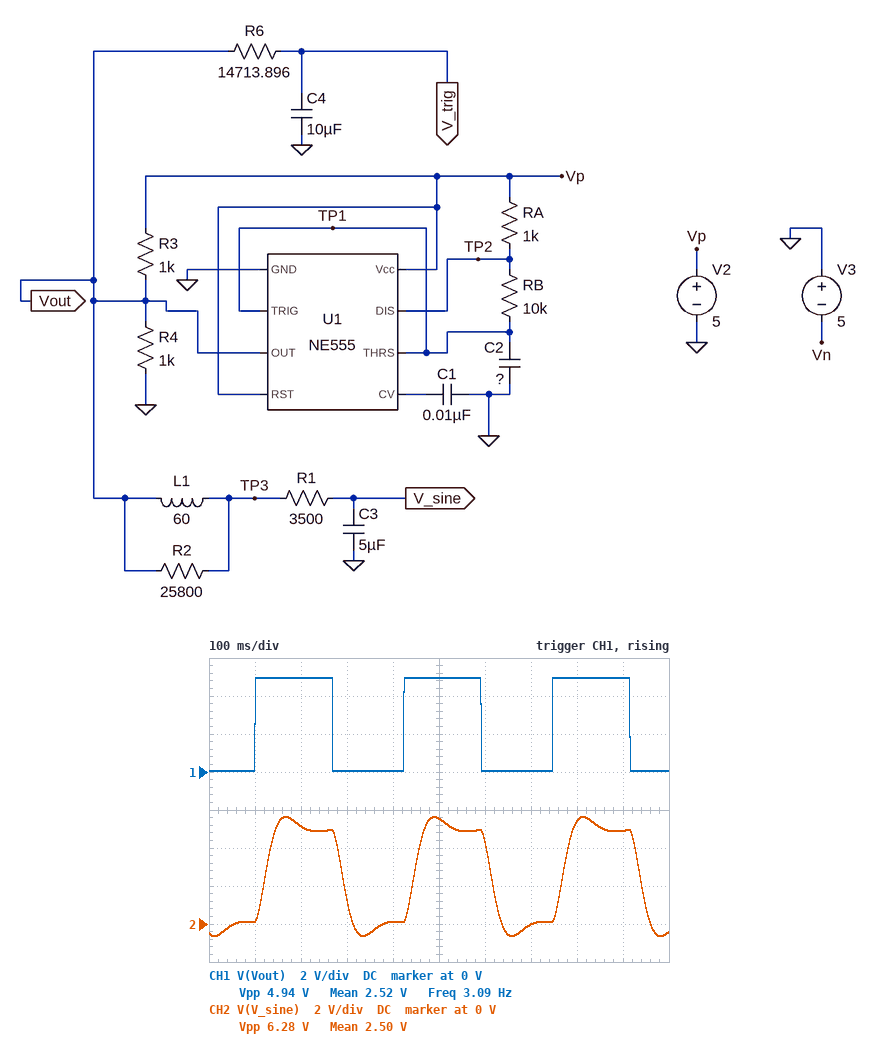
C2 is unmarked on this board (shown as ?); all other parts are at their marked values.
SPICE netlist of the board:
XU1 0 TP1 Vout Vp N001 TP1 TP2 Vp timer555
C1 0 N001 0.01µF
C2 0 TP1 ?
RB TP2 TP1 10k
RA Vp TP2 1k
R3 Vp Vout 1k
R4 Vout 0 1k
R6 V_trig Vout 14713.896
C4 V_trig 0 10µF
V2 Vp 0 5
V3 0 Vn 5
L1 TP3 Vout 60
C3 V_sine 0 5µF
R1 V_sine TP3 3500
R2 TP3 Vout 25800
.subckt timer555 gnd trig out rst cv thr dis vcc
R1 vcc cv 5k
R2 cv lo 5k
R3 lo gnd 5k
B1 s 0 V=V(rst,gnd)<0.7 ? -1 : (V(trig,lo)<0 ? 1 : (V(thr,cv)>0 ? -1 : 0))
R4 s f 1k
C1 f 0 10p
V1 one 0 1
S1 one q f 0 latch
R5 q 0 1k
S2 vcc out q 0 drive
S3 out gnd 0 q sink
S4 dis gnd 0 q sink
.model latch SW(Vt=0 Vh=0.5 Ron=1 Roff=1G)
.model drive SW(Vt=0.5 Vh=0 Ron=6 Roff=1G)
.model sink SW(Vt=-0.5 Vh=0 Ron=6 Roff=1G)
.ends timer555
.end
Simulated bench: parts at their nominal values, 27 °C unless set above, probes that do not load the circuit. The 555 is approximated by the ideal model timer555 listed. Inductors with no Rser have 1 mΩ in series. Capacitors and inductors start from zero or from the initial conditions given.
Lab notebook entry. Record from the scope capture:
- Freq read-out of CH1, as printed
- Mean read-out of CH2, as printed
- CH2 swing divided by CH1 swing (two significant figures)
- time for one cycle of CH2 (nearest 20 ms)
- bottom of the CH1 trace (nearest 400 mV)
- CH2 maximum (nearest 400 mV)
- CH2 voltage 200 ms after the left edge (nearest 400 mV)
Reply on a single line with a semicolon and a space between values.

3.09 Hz; 2.50 V; 1.3; 320 ms; 0 V; 5.6 V; 5.2 V
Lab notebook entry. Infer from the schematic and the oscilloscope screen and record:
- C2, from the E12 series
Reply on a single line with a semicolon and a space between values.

22 µF
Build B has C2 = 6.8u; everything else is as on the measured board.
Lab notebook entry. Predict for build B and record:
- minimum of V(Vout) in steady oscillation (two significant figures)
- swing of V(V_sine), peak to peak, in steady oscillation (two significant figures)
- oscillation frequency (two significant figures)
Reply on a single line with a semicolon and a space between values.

30 mV; 5.1 V; 10 Hz
